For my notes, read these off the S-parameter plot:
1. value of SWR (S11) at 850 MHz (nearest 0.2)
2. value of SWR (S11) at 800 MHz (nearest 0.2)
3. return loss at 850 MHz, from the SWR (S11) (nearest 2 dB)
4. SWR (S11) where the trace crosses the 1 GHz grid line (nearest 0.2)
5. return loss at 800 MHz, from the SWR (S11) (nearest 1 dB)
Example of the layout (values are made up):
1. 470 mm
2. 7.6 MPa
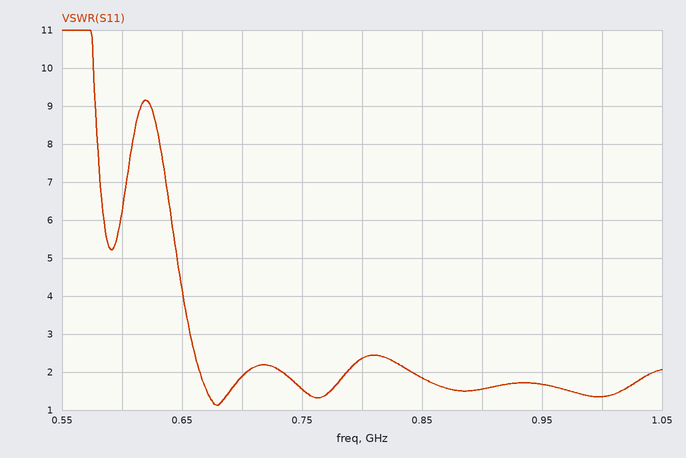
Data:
1. 1.8
2. 2.4
3. 10 dB
4. 1.4
5. 8 dB
